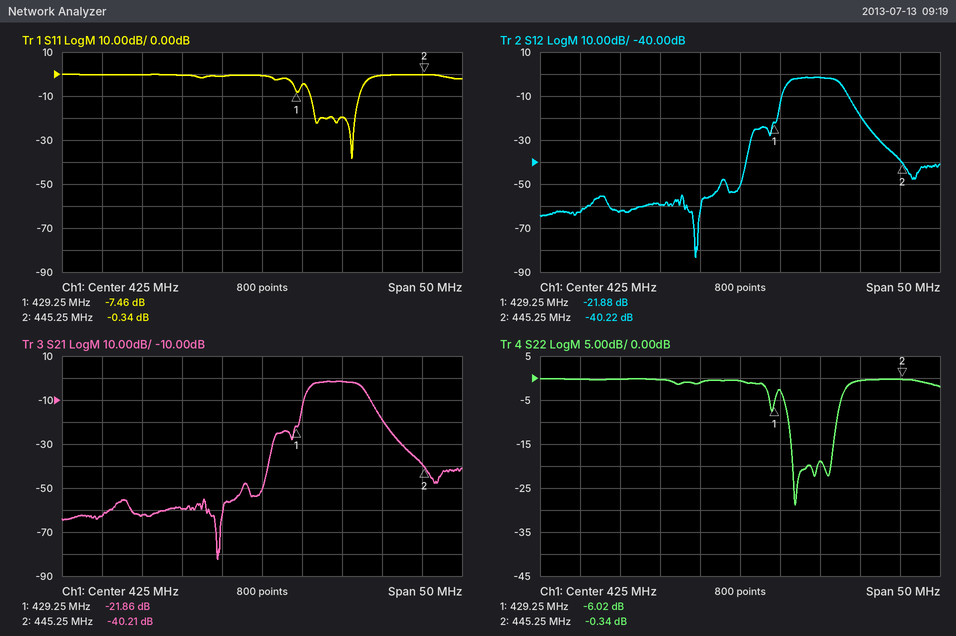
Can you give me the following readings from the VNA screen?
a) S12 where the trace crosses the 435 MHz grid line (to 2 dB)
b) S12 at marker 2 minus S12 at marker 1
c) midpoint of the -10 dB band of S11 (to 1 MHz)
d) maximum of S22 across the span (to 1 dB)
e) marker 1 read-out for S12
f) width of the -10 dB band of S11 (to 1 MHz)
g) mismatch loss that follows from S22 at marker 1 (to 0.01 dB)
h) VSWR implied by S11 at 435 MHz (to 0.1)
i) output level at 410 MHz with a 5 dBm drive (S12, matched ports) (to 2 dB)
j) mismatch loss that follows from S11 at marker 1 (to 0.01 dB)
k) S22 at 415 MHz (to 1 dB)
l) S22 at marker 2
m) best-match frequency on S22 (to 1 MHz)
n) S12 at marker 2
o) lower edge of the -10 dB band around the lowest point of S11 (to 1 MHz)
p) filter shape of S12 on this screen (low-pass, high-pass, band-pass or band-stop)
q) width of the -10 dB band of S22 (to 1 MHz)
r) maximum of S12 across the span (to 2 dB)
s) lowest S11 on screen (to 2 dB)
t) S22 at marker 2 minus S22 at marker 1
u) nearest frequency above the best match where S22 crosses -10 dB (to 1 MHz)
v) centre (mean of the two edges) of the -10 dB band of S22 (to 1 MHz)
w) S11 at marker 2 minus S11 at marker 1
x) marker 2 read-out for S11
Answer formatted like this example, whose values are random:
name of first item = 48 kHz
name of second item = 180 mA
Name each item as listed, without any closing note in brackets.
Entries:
S12 where the trace crosses the 435 MHz grid line = -2 dB
S12 at marker 2 minus S12 at marker 1 = -18.34 dB
midpoint of the -10 dB band of S11 = 434 MHz
maximum of S22 across the span = 0 dB
marker 1 read-out for S12 = -21.88 dB
width of the -10 dB band of S11 = 6 MHz
mismatch loss that follows from S22 at marker 1 = 1.25 dB
VSWR implied by S11 at 435 MHz = 1.2
output level at 410 MHz with a 5 dBm drive (S12, matched ports) = -58 dBm
mismatch loss that follows from S11 at marker 1 = 0.86 dB
S22 at 415 MHz = 0 dB
S22 at marker 2 = -0.34 dB
best-match frequency on S22 = 432 MHz
S12 at marker 2 = -40.22 dB
lower edge of the -10 dB band around the lowest point of S11 = 431 MHz
filter shape of S12 on this screen = band-pass
width of the -10 dB band of S22 = 6 MHz
maximum of S12 across the span = -2 dB
lowest S11 on screen = -38 dB
S22 at marker 2 minus S22 at marker 1 = 5.68 dB
nearest frequency above the best match where S22 crosses -10 dB = 437 MHz
centre (mean of the two edges) of the -10 dB band of S22 = 434 MHz
S11 at marker 2 minus S11 at marker 1 = 7.12 dB
marker 2 read-out for S11 = -0.34 dB
